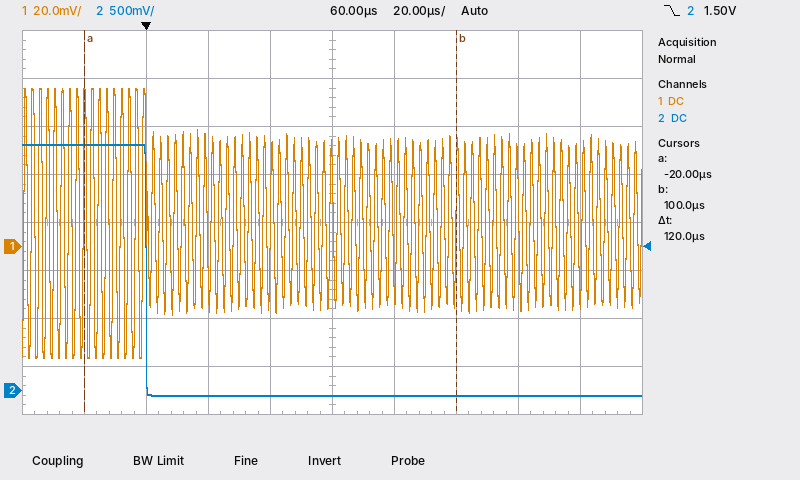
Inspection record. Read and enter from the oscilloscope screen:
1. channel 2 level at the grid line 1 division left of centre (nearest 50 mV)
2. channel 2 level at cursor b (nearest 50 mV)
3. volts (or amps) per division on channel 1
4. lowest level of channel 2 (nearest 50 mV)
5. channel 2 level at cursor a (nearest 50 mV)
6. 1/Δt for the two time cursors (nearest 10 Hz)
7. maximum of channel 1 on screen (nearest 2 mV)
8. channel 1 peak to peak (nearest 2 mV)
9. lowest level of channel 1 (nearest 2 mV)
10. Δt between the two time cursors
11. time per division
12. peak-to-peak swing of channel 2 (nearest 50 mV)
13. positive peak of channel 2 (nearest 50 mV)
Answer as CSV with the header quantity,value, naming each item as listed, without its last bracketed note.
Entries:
quantity,value
channel 2 level at the grid line 1 division left of centre,-50 mV
channel 2 level at cursor b,-50 mV
volts (or amps) per division on channel 1,20 mV
lowest level of channel 2,-50 mV
channel 2 level at cursor a,2.55 V
1/Δt for the two time cursors,8.33 kHz
maximum of channel 1 on screen,66 mV
channel 1 peak to peak,112 mV
lowest level of channel 1,-46 mV
Δt between the two time cursors,120 µs
time per division,20 µs
peak-to-peak swing of channel 2,2.60 V
positive peak of channel 2,2.55 V
